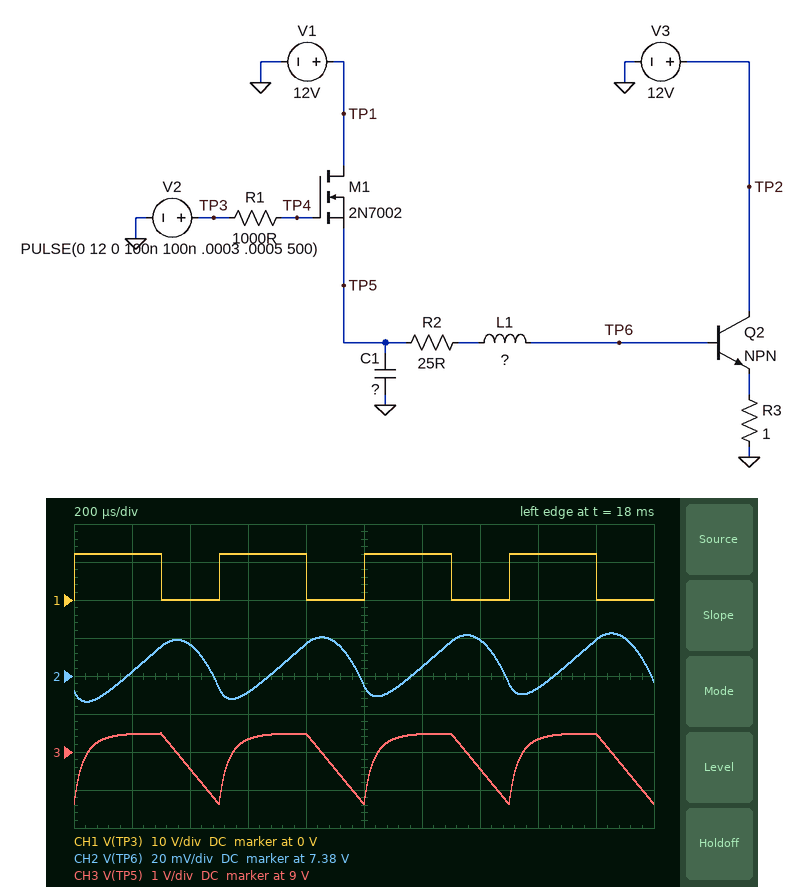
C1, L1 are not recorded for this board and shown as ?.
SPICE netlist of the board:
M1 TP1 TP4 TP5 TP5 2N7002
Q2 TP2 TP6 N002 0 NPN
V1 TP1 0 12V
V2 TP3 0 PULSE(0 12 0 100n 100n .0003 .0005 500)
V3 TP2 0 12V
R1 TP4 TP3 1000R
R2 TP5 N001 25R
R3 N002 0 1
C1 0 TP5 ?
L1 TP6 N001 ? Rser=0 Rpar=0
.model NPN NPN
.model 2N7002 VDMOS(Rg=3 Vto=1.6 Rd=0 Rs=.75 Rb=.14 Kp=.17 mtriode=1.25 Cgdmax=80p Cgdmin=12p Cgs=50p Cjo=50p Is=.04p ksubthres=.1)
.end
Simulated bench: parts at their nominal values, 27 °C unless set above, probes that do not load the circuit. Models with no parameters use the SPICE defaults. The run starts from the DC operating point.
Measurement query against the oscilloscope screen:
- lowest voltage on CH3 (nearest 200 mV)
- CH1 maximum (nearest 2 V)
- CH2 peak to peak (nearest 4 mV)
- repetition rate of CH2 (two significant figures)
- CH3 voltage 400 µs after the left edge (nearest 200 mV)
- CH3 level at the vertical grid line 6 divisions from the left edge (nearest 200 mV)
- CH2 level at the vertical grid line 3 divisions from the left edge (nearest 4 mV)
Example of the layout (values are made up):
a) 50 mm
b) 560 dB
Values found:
a) 7.6 V
b) 12 V
c) 36 mV
d) 2.0 kHz
e) 8.6 V
f) 9.4 V
g) 7.372 V
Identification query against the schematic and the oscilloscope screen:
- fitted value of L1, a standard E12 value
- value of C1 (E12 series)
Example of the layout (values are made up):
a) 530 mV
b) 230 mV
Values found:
a) 390 mH
b) 6.8 µF
